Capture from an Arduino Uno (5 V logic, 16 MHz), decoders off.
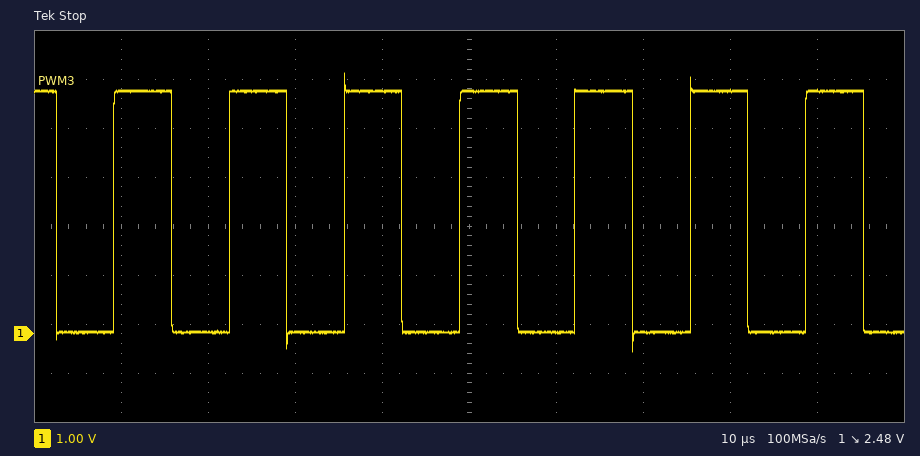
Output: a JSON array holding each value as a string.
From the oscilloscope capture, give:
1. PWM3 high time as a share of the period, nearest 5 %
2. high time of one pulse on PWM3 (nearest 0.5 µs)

["50 %", "6.5 µs"]
